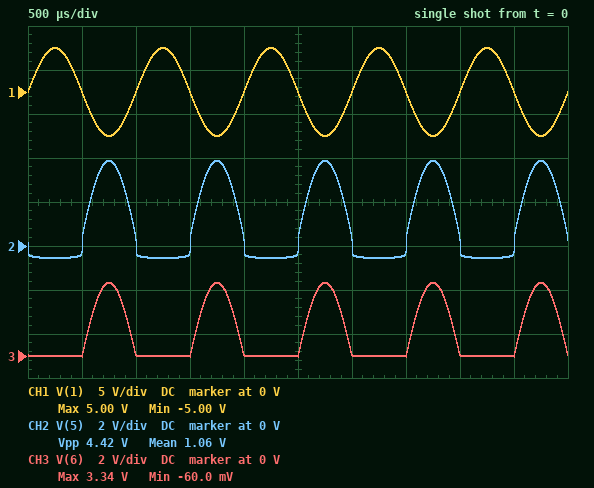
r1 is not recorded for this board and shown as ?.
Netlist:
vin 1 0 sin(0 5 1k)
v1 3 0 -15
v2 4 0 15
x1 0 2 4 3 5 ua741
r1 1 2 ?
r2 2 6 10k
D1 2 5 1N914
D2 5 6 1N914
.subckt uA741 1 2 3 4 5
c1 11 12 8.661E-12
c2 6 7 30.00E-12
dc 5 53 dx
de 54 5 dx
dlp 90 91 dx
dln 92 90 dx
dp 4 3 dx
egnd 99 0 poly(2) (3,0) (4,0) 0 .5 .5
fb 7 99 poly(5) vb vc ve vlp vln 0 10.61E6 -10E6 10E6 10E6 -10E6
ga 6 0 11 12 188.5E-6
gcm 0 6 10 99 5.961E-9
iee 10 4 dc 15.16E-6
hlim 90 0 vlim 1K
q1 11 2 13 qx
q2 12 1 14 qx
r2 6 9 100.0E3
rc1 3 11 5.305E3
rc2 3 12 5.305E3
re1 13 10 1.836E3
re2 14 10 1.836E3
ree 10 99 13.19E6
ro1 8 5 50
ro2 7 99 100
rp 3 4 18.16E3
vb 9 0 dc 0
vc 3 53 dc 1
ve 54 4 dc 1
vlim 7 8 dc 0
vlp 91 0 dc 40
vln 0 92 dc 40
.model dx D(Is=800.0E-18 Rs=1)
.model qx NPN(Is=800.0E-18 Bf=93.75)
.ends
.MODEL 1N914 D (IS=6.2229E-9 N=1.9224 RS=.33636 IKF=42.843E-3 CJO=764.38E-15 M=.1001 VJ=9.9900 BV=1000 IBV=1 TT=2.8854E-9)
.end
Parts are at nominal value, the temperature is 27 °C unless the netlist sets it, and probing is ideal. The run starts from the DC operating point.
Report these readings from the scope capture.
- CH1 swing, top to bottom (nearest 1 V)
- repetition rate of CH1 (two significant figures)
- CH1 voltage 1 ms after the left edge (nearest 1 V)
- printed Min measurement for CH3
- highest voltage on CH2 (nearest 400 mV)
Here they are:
10 V
1.0 kHz
0 V
-60.0 mV
4.0 V
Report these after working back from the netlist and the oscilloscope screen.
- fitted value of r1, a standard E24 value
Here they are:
15 kΩ
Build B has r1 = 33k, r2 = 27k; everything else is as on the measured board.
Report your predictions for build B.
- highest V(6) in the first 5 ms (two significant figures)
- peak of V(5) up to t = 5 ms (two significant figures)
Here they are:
4.1 V
4.6 V
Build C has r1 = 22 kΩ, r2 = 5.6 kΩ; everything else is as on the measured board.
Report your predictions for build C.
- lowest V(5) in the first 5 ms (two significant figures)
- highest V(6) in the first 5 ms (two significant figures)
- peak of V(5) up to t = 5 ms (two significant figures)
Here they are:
-530 mV
1.3 V
1.8 V
